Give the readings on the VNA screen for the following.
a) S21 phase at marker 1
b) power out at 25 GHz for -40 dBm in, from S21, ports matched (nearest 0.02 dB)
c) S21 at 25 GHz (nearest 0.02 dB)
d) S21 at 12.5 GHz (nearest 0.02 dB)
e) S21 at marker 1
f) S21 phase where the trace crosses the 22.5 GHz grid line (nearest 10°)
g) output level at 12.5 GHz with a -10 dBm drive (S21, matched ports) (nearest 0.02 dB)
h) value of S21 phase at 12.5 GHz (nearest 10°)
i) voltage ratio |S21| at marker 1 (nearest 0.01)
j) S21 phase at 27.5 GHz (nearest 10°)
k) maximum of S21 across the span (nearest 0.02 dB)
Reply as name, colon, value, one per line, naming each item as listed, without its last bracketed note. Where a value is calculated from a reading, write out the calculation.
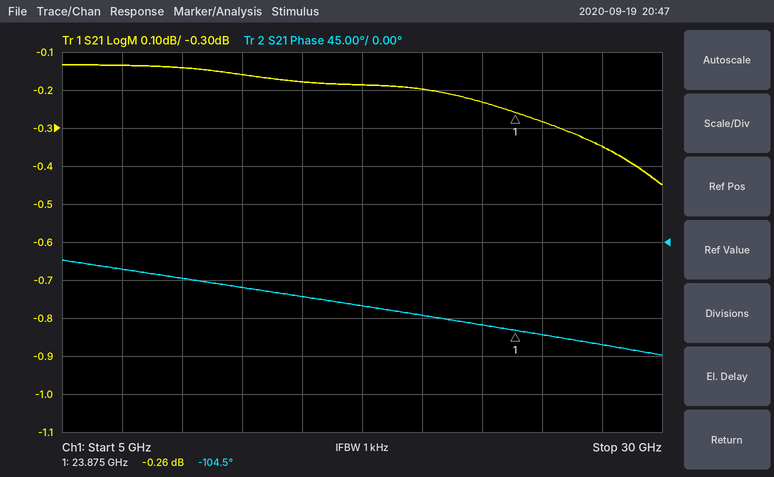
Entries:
S21 phase at marker 1: -104.5°
power out at 25 GHz for -40 dBm in, from S21, ports matched: -40 dBm + (-0.28 dB) = -40.28 dBm
S21 at 25 GHz: -0.28 dB
S21 at 12.5 GHz: -0.16 dB
S21 at marker 1: -0.26 dB
S21 phase where the trace crosses the 22.5 GHz grid line: -100°
output level at 12.5 GHz with a -10 dBm drive (S21, matched ports): -10 dBm + (-0.16 dB) = -10.16 dBm
value of S21 phase at 12.5 GHz: -50°
voltage ratio |S21| at marker 1: 10^(-0.26/20) ≈ 0.97
S21 phase at 27.5 GHz: -120°
maximum of S21 across the span: -0.14 dB
